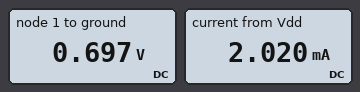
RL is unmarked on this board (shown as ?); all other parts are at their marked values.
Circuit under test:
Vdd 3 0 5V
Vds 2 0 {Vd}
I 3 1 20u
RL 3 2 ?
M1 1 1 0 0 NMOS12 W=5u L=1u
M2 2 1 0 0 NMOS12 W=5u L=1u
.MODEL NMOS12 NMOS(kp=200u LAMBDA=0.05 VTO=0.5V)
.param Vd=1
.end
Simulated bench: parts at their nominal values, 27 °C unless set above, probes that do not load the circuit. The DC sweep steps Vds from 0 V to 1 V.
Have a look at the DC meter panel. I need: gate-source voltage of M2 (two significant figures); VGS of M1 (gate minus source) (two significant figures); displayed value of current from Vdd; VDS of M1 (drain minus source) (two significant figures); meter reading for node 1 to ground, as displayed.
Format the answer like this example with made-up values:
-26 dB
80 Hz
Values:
700 mV
700 mV
2.020 mA
700 mV
0.697 V
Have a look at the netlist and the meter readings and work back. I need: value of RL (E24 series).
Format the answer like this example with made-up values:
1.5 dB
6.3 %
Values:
2 kΩ
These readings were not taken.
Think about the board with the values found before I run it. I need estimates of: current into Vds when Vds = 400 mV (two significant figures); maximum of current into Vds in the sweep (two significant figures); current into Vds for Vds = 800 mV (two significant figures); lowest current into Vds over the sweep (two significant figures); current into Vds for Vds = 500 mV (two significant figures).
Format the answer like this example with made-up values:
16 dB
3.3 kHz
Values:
2.3 mA
2.5 mA
2.1 mA
2.0 mA
2.2 mA
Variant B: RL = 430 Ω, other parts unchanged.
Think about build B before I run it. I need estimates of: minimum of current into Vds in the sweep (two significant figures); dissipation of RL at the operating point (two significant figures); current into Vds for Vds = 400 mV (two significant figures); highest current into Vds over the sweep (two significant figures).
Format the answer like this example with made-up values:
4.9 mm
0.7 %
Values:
9.3 mA
37 mW
11 mA
12 mA
